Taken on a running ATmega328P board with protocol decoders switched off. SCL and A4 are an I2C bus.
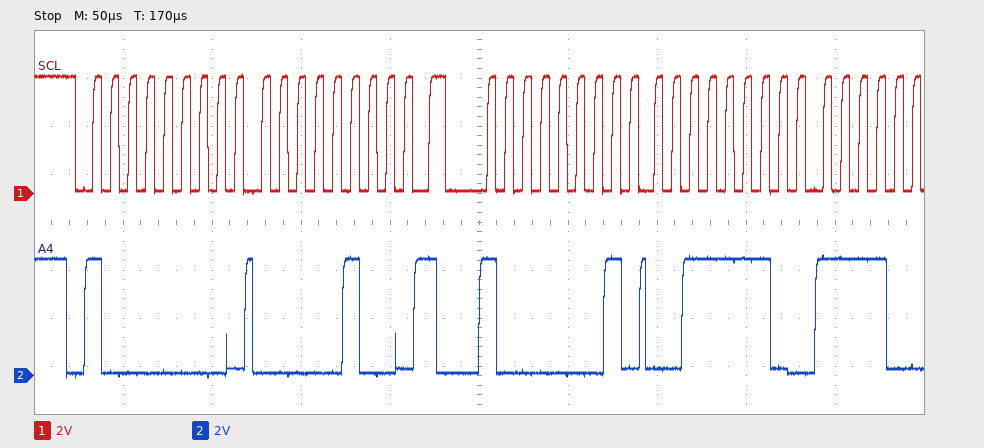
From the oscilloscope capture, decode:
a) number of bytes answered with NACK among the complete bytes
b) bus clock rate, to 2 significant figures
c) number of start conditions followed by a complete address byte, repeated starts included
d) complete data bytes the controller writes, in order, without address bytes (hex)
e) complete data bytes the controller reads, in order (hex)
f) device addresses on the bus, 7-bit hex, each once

0
100 kHz
2
04
3E
0x40
